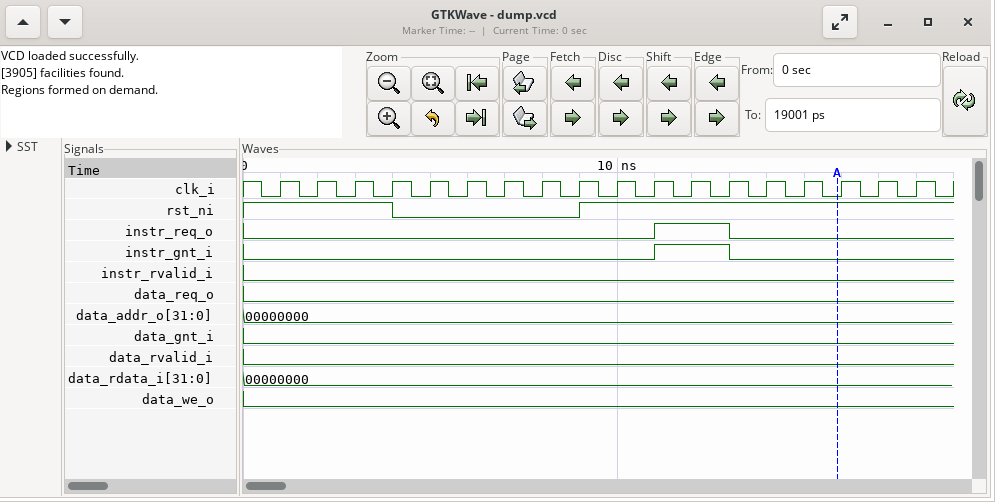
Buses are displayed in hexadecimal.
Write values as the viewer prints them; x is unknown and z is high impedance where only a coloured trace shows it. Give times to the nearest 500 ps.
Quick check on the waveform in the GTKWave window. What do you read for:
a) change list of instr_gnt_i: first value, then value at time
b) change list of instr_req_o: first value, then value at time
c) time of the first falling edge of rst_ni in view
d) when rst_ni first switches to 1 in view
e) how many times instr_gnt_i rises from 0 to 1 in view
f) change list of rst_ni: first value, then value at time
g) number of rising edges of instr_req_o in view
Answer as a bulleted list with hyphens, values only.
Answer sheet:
- 0, 1 at 11000 ps, 0 at 13000 ps
- 0, 1 at 11000 ps, 0 at 13000 ps
- 4000 ps
- 9000 ps
- 1
- 1, 0 at 4000 ps, 1 at 9000 ps
- 1
